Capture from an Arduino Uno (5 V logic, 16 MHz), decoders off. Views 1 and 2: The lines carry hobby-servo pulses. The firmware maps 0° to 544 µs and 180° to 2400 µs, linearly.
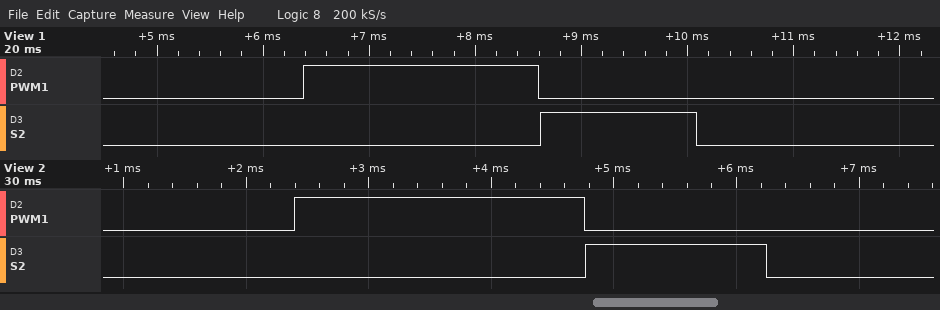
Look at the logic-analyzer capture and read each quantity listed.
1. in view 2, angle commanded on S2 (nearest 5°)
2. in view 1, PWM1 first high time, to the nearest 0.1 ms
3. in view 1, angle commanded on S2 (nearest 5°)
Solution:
90°
2.2 ms
90°
